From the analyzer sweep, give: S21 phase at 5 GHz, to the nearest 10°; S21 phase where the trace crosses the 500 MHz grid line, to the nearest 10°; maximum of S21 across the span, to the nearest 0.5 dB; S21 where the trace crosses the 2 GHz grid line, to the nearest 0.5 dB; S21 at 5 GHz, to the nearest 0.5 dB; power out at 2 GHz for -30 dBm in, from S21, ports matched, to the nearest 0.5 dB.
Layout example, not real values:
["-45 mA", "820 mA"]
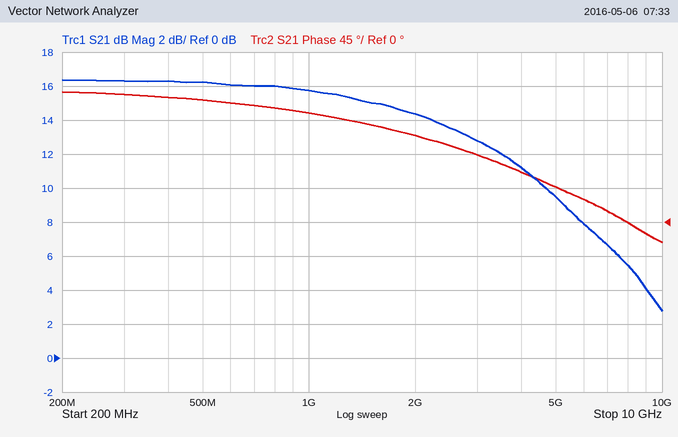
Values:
["50°", "160°", "16.5 dB", "14.5 dB", "9.5 dB", "-15.5 dBm"]
